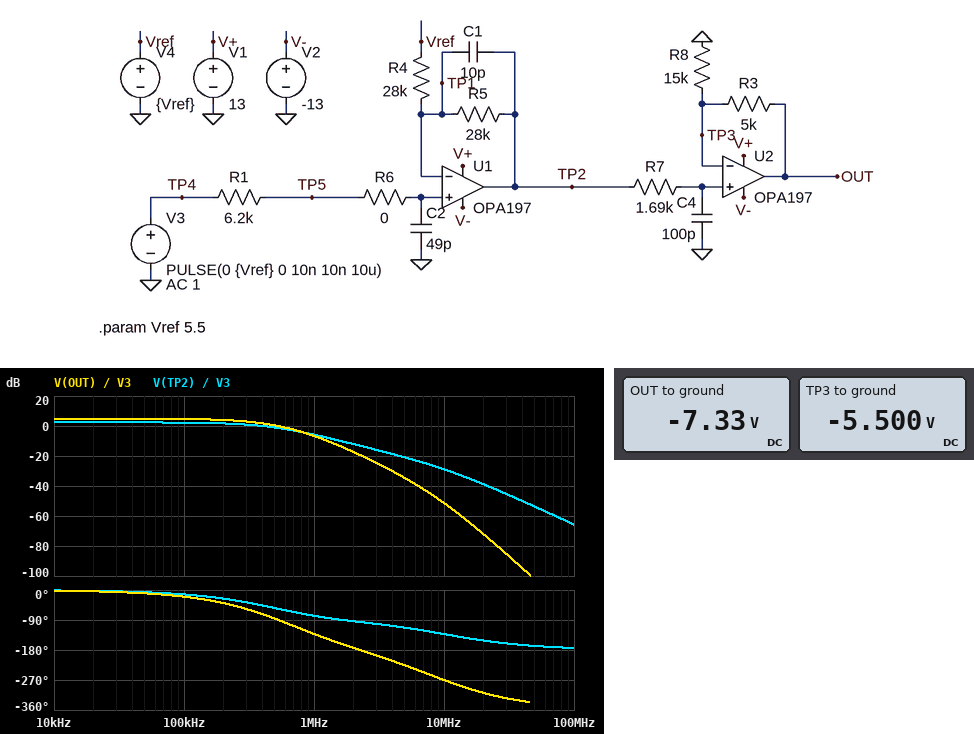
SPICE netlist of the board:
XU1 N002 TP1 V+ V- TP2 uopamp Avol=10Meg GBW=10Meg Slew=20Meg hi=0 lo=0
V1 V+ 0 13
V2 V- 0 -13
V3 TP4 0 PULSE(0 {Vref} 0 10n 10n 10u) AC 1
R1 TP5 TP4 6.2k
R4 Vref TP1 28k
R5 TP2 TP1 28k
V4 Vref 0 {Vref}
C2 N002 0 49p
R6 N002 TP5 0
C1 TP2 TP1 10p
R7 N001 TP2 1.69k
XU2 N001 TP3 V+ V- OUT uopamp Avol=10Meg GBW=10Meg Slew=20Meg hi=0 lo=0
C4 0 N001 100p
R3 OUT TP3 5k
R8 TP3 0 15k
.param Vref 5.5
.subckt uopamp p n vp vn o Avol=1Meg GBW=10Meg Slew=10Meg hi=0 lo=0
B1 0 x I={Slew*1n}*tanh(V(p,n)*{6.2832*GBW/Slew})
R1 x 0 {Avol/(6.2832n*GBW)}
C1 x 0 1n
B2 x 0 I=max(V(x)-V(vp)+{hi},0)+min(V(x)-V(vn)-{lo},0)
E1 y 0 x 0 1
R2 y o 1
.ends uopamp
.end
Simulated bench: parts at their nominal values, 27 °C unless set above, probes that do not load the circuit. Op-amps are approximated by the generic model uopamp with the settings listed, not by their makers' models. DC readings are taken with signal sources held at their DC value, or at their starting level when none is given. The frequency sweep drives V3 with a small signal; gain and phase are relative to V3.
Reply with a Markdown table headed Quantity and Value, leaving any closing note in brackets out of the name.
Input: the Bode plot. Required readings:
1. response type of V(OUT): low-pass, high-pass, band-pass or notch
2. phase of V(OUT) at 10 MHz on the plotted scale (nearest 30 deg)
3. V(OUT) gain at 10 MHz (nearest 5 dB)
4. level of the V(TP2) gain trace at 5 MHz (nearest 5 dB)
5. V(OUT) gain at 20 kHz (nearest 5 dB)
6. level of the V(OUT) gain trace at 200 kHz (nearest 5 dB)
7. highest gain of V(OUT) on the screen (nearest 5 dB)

| Quantity | Value |
|---|---|
| response type of V(OUT): low-pass, high-pass, band-pass or notch | low-pass |
| phase of V(OUT) at 10 MHz on the plotted scale | -270 deg |
| V(OUT) gain at 10 MHz | -50 dB |
| level of the V(TP2) gain trace at 5 MHz | -20 dB |
| V(OUT) gain at 20 kHz | 5 dB |
| level of the V(OUT) gain trace at 200 kHz | 5 dB |
| highest gain of V(OUT) on the screen | 5 dB |
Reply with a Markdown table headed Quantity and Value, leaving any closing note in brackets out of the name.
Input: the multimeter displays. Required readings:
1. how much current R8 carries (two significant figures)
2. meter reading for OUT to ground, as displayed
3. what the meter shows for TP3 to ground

| Quantity | Value |
|---|---|
| how much current R8 carries | 370 µA |
| meter reading for OUT to ground, as displayed | -7.33 V |
| what the meter shows for TP3 to ground | -5.500 V |
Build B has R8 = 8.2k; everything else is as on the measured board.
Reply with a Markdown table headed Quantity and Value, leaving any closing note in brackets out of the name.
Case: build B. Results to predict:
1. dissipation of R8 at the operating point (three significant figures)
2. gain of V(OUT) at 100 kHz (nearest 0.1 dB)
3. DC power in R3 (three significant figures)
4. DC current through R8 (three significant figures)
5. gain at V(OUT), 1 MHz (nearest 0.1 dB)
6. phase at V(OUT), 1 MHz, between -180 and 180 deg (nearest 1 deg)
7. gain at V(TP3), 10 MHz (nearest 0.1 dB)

| Quantity | Value |
|---|---|
| dissipation of R8 at the operating point | 3.69 mW |
| gain of V(OUT) at 100 kHz | 6.3 dB |
| DC power in R3 | 2.25 mW |
| DC current through R8 | 671 µA |
| gain at V(OUT), 1 MHz | -5.0 dB |
| phase at V(OUT), 1 MHz, between -180 and 180 deg | -133 deg |
| gain at V(TP3), 10 MHz | -55.0 dB |
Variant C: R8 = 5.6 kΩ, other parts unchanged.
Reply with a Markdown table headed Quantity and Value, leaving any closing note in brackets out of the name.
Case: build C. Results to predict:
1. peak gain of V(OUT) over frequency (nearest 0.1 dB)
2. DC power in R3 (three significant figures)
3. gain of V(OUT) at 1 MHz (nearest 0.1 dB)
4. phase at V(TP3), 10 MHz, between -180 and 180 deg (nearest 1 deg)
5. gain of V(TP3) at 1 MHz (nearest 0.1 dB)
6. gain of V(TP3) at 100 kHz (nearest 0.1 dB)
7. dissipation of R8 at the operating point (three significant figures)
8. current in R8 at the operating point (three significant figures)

| Quantity | Value |
|---|---|
| peak gain of V(OUT) over frequency | 8.0 dB |
| DC power in R3 | 4.82 mW |
| gain of V(OUT) at 1 MHz | -3.7 dB |
| phase at V(TP3), 10 MHz, between -180 and 180 deg | 81 deg |
| gain of V(TP3) at 1 MHz | -9.2 dB |
| gain of V(TP3) at 100 kHz | 2.2 dB |
| dissipation of R8 at the operating point | 5.40 mW |
| current in R8 at the operating point | 982 µA |
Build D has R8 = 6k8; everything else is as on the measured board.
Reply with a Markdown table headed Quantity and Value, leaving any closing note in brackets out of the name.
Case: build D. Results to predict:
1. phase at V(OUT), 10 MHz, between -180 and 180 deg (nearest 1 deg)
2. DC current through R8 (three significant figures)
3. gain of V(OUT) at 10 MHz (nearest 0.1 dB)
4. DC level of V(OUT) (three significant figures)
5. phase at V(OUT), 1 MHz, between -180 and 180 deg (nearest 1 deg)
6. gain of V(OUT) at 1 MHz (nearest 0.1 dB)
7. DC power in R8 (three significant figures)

| Quantity | Value |
|---|---|
| phase at V(OUT), 10 MHz, between -180 and 180 deg | 83 deg |
| DC current through R8 | 809 µA |
| gain of V(OUT) at 10 MHz | -50.7 dB |
| DC level of V(OUT) | -9.54 V |
| phase at V(OUT), 1 MHz, between -180 and 180 deg | -134 deg |
| gain of V(OUT) at 1 MHz | -4.4 dB |
| DC power in R8 | 4.45 mW |
